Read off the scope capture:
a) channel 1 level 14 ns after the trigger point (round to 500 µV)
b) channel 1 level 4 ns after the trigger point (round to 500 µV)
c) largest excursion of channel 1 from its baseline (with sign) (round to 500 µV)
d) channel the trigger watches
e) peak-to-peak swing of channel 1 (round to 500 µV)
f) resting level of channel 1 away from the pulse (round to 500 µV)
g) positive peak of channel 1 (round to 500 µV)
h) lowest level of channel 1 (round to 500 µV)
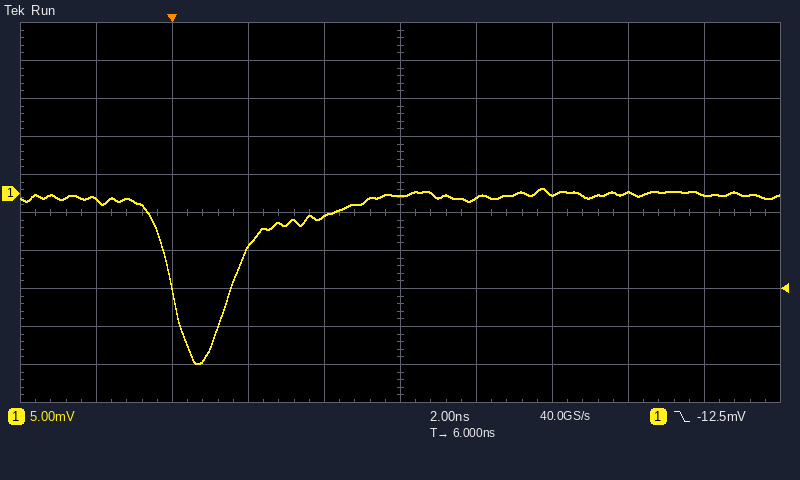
0.0 mV
-3.0 mV
-22.0 mV
channel 1
23.0 mV
-500 µV
500 µV
-22.5 mV
